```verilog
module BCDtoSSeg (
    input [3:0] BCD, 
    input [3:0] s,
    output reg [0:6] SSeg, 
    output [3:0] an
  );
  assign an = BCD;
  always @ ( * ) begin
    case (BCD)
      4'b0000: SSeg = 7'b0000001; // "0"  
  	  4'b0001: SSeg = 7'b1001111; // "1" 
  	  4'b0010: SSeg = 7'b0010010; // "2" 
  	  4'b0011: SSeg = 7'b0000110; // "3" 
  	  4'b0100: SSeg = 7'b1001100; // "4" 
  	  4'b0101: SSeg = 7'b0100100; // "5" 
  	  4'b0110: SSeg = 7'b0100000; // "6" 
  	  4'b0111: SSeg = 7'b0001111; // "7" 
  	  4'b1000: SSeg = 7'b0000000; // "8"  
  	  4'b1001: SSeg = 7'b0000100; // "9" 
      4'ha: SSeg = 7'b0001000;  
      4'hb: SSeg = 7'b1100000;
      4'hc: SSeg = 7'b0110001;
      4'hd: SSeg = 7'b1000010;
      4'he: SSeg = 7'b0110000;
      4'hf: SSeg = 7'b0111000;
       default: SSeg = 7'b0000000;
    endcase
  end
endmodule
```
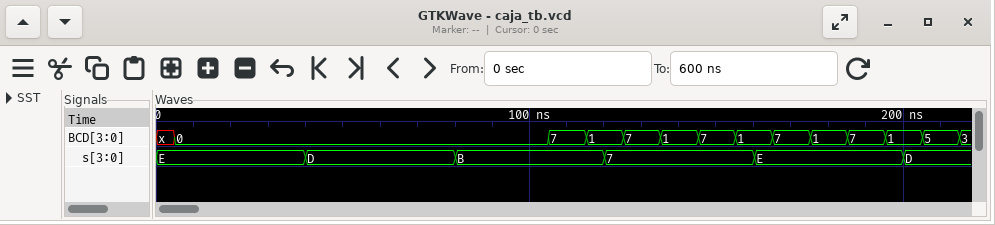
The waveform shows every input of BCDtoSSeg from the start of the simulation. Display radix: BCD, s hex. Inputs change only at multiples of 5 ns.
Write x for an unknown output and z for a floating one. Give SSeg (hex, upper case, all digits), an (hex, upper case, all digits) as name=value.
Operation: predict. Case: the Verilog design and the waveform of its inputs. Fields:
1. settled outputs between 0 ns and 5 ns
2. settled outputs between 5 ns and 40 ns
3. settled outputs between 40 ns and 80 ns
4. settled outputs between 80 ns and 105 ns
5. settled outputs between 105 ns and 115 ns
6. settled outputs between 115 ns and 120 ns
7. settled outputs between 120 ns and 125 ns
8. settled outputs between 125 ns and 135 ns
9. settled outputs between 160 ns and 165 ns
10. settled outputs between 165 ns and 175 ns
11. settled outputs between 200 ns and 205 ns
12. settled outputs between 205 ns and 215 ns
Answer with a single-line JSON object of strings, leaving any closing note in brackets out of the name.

{"settled outputs between 0 ns and 5 ns": "SSeg=x, an=x", "settled outputs between 5 ns and 40 ns": "SSeg=01, an=0", "settled outputs between 40 ns and 80 ns": "SSeg=01, an=0", "settled outputs between 80 ns and 105 ns": "SSeg=01, an=0", "settled outputs between 105 ns and 115 ns": "SSeg=0F, an=7", "settled outputs between 115 ns and 120 ns": "SSeg=4F, an=1", "settled outputs between 120 ns and 125 ns": "SSeg=4F, an=1", "settled outputs between 125 ns and 135 ns": "SSeg=0F, an=7", "settled outputs between 160 ns and 165 ns": "SSeg=4F, an=1", "settled outputs between 165 ns and 175 ns": "SSeg=0F, an=7", "settled outputs between 200 ns and 205 ns": "SSeg=4F, an=1", "settled outputs between 205 ns and 215 ns": "SSeg=24, an=5"}
